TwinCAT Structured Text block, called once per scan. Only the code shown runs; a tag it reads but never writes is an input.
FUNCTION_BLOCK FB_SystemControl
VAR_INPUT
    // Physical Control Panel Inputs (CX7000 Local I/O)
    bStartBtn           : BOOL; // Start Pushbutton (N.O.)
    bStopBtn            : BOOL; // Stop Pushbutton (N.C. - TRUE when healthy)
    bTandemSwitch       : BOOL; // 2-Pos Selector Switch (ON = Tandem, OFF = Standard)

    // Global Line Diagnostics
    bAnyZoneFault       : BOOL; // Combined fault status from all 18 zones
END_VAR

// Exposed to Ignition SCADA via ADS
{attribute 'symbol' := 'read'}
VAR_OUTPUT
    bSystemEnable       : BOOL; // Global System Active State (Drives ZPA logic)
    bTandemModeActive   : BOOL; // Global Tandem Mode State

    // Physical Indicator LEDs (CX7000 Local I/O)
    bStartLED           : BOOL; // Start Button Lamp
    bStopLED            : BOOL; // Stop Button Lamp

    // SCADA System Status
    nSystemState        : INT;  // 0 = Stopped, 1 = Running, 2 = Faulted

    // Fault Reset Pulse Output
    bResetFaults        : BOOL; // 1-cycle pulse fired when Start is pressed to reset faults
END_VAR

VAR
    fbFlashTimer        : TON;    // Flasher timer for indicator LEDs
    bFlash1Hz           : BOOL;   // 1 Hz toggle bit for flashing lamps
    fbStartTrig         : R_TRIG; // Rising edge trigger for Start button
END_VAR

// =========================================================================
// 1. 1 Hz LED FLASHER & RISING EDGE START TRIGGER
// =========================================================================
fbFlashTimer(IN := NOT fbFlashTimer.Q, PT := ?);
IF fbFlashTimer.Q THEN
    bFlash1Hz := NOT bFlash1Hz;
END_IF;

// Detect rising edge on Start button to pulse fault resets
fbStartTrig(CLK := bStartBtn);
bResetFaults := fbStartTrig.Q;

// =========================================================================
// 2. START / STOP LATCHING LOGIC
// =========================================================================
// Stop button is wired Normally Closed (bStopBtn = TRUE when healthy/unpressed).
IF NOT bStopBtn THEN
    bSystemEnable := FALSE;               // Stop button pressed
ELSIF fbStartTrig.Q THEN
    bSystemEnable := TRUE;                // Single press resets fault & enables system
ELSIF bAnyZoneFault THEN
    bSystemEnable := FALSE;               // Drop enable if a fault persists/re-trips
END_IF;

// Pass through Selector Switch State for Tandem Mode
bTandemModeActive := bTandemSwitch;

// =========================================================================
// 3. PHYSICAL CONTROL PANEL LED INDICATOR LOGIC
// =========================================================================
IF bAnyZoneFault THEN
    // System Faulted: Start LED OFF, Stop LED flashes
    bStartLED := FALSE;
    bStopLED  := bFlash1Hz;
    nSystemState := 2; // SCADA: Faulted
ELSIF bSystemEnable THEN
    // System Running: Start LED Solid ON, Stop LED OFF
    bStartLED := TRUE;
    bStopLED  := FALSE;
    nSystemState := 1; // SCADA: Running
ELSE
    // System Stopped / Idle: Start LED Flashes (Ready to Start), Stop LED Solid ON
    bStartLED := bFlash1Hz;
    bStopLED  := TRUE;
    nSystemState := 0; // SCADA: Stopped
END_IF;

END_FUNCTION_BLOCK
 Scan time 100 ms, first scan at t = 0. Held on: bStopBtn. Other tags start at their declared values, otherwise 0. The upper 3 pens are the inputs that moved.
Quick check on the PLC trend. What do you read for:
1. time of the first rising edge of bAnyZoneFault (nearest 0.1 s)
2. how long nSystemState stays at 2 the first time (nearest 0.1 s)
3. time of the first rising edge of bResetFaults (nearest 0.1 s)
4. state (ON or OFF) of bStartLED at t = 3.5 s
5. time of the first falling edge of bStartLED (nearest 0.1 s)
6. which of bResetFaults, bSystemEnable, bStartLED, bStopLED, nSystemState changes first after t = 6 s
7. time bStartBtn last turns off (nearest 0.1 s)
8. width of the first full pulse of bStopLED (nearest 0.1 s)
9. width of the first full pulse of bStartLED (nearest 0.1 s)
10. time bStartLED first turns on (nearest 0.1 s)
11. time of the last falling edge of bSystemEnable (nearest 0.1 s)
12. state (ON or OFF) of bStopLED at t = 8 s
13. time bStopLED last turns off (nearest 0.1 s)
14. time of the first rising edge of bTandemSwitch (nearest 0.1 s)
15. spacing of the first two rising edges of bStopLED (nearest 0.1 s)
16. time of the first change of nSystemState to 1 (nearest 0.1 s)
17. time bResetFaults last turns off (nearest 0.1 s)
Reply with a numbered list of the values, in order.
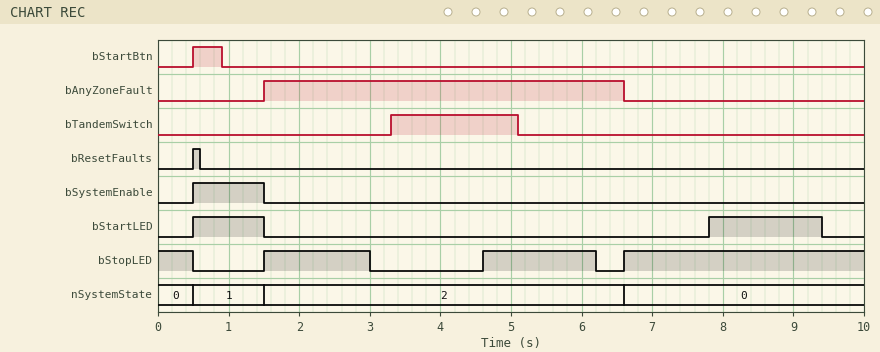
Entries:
1. 1.5 s
2. 5.1 s
3. 0.5 s
4. OFF
5. 1.5 s
6. bStopLED
7. 0.9 s
8. 1.5 s
9. 1.0 s
10. 0.5 s
11. 1.5 s
12. ON
13. 6.2 s
14. 3.3 s
15. 3.1 s
16. 0.5 s
17. 0.6 s
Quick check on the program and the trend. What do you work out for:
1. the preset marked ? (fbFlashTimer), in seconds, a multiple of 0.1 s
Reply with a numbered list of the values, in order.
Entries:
1. 1.4 s
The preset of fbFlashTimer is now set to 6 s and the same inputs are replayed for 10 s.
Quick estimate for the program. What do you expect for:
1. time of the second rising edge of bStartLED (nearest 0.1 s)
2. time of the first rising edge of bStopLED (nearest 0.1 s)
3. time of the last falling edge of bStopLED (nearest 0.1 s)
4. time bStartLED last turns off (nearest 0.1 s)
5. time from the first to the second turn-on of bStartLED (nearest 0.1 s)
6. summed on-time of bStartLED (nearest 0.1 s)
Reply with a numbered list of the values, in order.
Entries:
1. 6.6 s
2. 6.0 s
3. 0.5 s
4. 1.5 s
5. 6.1 s
6. 4.4 s
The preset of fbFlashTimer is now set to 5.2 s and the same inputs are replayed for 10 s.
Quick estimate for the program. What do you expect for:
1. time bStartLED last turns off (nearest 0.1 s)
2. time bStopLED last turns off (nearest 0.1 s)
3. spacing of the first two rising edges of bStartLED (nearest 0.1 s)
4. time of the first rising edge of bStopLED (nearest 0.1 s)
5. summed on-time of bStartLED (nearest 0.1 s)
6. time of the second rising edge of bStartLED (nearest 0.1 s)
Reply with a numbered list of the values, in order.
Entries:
1. 1.5 s
2. 0.5 s
3. 6.1 s
4. 5.2 s
5. 4.4 s
6. 6.6 s
